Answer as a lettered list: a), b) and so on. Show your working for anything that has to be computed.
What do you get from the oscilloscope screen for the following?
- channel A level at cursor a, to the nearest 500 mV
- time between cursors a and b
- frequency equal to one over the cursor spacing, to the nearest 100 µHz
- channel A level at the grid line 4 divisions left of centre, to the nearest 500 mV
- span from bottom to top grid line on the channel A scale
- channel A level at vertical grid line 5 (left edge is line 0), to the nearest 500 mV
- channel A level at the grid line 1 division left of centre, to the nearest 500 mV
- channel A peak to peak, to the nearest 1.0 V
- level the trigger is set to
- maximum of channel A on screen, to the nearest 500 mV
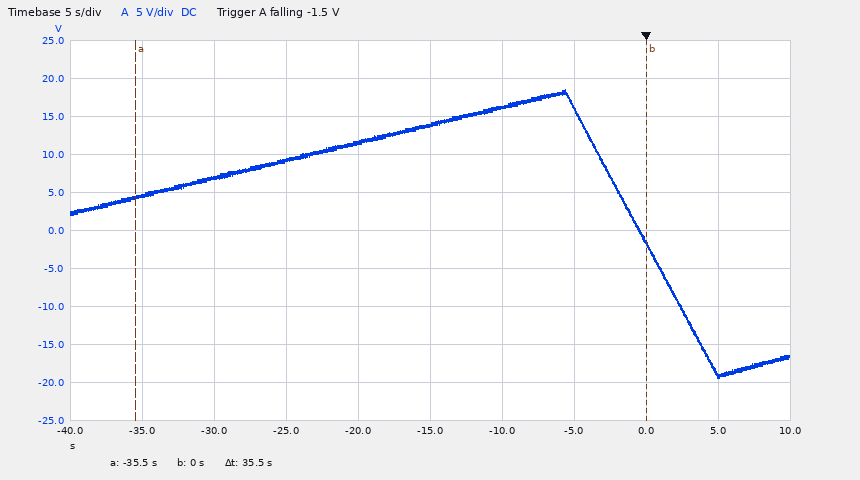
a) 4.5 V
b) 35.5 s
c) 1 / 35.5 s ≈ 28.2 mHz
d) 4.5 V
e) 50 V
f) 14.0 V
g) 11.5 V
h) 38.0 V
i) -1.5 V
j) 18.5 V
